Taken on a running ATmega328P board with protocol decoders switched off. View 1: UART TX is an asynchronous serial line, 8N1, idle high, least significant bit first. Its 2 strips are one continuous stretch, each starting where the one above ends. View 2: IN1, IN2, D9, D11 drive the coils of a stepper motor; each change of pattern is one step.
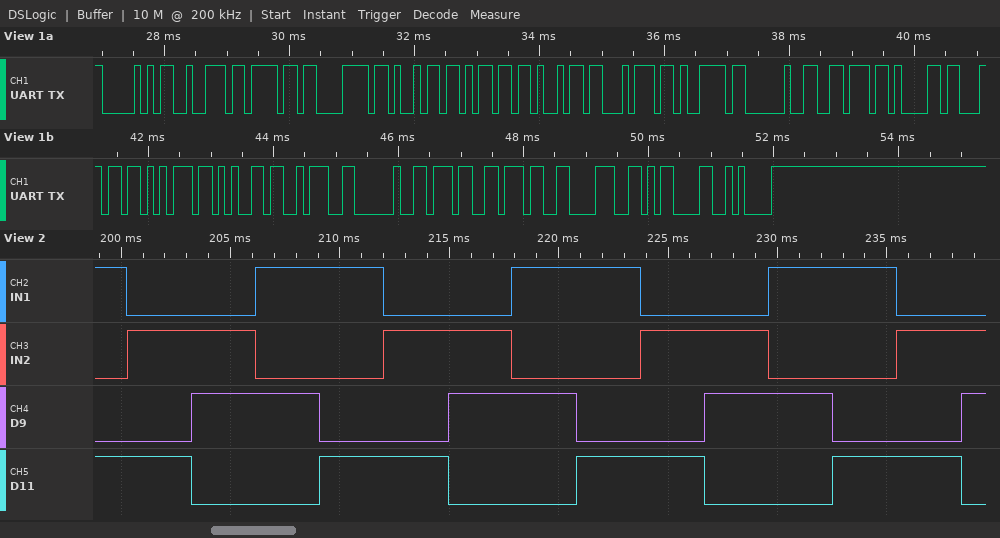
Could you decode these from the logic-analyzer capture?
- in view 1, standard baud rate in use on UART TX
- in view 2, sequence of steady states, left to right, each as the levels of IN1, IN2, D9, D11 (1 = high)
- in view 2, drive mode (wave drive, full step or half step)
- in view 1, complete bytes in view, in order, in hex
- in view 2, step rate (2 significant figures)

9600 baud
1001 0101 0110 1010 1001 0101 0110 1010 1001 0101 0110 1010 1001 0101 0110
full step
50 72 6F 78 69 6D 69 74 79 20 76 61 6C 75 65 3A 20 37 37 38 0D 0A
340 steps/s
